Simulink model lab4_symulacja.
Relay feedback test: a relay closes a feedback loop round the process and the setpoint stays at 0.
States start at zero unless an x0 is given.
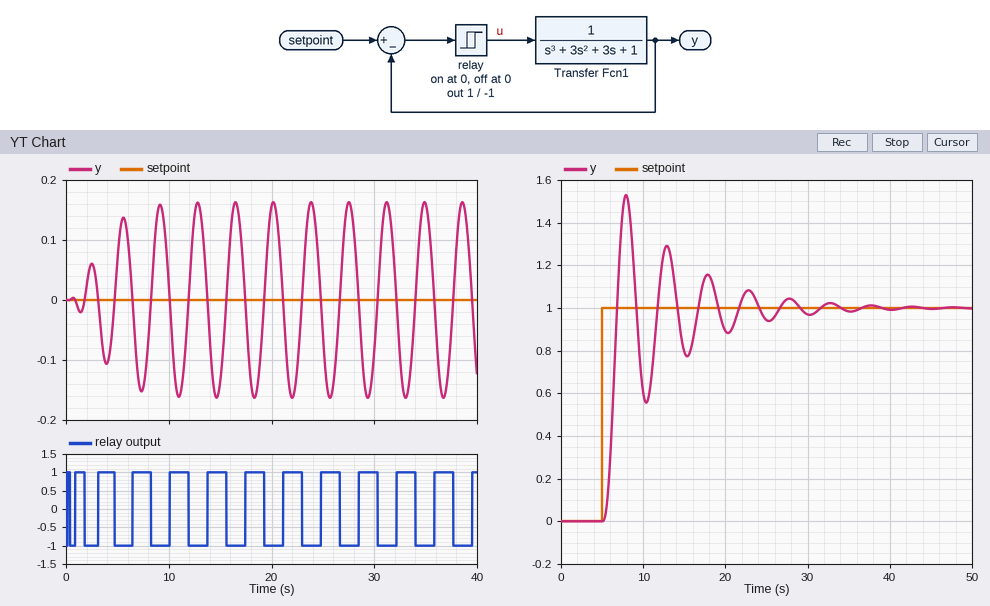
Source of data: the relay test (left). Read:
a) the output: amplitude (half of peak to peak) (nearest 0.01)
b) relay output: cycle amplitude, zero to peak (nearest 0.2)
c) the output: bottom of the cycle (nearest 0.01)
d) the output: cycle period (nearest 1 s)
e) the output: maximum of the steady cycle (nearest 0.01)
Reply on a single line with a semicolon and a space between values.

0.16; 1.0; -0.16; 4 s; 0.16
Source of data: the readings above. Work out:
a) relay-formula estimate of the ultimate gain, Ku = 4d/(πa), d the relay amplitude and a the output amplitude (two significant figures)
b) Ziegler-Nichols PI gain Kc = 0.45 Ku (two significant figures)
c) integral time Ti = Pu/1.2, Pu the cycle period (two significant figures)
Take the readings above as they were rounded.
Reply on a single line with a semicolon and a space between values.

8.0; 3.6; 3.3 s
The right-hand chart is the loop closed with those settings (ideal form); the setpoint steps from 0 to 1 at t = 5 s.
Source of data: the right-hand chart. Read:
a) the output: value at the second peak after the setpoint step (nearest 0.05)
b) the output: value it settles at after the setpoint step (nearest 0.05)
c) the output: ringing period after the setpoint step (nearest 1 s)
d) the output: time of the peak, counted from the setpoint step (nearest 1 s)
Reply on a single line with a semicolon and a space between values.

1.30; 1.00; 5 s; 3 s
